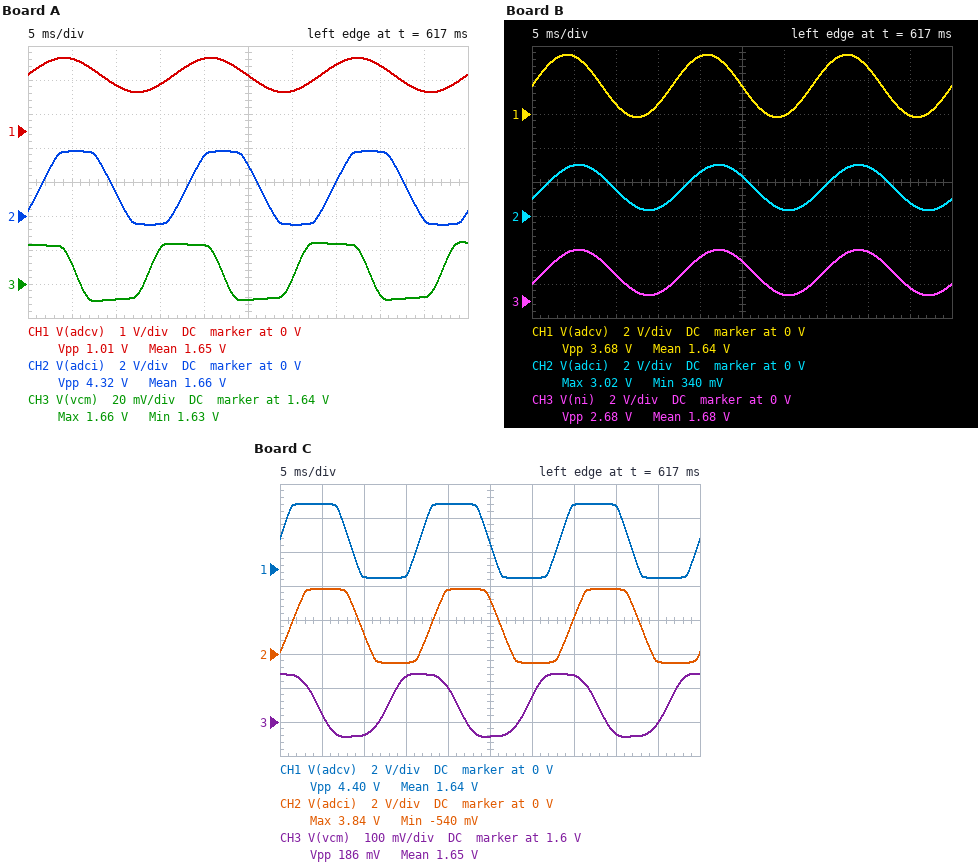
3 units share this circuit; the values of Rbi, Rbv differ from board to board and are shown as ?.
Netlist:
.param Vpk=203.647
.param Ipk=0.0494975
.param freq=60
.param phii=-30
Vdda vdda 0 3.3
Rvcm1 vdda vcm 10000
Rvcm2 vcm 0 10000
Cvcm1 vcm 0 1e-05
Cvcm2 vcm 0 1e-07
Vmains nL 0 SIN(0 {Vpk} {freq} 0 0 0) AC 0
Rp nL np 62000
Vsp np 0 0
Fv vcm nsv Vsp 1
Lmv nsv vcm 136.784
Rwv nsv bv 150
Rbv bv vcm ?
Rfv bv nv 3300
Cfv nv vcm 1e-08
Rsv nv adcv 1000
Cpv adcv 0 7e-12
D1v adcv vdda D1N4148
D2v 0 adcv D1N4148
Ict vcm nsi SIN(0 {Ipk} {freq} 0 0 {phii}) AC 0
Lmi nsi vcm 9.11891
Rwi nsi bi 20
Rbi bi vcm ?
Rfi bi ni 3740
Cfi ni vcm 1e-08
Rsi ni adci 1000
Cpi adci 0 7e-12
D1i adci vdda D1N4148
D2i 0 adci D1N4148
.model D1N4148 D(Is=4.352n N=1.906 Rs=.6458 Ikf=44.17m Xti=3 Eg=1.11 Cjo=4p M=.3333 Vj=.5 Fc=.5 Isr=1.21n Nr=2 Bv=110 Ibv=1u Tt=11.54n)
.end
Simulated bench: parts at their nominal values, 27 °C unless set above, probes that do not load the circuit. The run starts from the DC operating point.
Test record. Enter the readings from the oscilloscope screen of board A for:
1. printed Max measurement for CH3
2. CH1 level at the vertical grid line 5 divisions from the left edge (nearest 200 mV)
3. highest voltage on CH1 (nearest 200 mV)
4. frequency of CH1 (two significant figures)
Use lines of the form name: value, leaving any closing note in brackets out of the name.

printed Max measurement for CH3: 1.66 V
CH1 level at the vertical grid line 5 divisions from the left edge: 1.6 V
highest voltage on CH1: 2.2 V
frequency of CH1: 60 Hz
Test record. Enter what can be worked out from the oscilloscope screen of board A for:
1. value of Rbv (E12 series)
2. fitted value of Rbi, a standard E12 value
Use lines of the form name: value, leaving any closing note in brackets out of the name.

value of Rbv: 150 Ω
fitted value of Rbi, a standard E12 value: 56 Ω
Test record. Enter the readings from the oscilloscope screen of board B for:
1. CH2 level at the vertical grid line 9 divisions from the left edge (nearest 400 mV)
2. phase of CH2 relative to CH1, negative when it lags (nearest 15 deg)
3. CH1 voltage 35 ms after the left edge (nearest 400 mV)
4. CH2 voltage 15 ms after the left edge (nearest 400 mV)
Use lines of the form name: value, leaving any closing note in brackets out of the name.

CH2 level at the vertical grid line 9 divisions from the left edge: 800 mV
phase of CH2 relative to CH1, negative when it lags: -30 deg
CH1 voltage 35 ms after the left edge: 2.8 V
CH2 voltage 15 ms after the left edge: 400 mV
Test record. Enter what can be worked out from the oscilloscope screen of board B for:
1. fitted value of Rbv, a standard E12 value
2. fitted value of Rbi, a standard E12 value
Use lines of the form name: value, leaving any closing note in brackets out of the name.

fitted value of Rbv, a standard E12 value: 560 Ω
fitted value of Rbi, a standard E12 value: 27 Ω
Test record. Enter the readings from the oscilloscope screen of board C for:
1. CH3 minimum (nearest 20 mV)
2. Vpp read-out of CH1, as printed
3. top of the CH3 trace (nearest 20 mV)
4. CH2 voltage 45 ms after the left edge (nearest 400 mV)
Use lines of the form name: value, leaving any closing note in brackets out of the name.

CH3 minimum: 1.56 V
Vpp read-out of CH1, as printed: 4.40 V
top of the CH3 trace: 1.74 V
CH2 voltage 45 ms after the left edge: -400 mV
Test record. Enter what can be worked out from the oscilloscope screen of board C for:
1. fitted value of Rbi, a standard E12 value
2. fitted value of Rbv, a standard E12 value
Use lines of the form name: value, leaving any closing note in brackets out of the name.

fitted value of Rbi, a standard E12 value: 68 Ω
fitted value of Rbv, a standard E12 value: 1.2 kΩ
